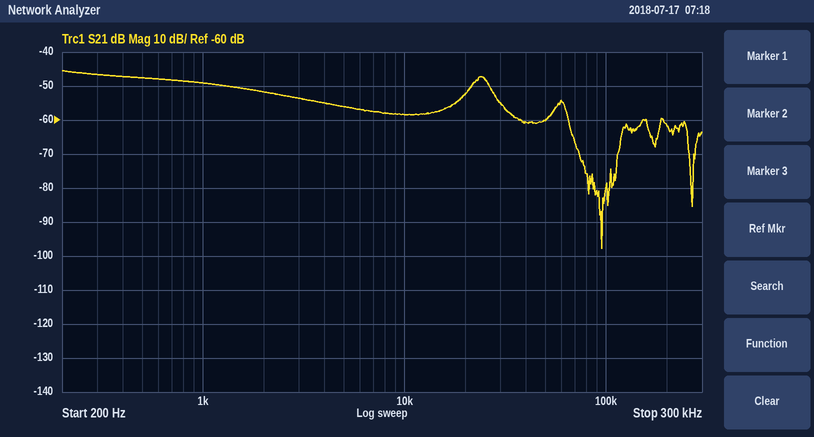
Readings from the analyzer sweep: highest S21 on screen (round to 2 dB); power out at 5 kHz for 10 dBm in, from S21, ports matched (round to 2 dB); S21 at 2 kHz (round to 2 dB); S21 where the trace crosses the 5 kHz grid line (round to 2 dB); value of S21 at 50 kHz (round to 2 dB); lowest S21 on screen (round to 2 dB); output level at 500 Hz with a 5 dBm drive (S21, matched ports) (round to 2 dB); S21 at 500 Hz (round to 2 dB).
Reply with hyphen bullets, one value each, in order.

- -46 dB
- -46 dBm
- -52 dB
- -56 dB
- -60 dB
- -98 dB
- -42 dBm
- -48 dB
